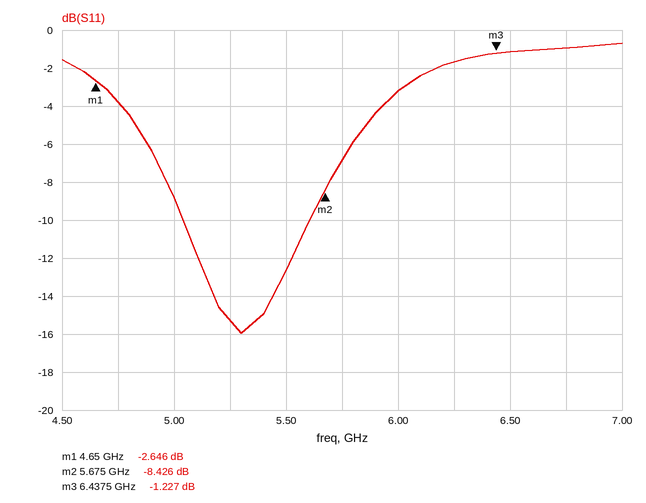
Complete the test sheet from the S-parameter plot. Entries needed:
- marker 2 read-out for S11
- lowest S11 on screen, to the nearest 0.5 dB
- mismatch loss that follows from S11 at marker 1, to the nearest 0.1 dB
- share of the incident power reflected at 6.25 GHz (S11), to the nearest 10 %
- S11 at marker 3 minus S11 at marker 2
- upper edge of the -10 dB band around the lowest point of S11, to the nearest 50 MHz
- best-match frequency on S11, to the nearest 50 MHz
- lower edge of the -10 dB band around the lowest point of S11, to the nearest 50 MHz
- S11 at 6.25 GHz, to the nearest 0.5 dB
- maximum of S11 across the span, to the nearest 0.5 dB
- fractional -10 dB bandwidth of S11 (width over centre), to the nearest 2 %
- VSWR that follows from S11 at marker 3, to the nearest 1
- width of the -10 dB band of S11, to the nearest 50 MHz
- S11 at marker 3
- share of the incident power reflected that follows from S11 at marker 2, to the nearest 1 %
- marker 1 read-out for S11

-8.426 dB
-16.0 dB
3.4 dB
70 %
7.199 dB
5.60 GHz
5.30 GHz
5.05 GHz
-1.5 dB
-0.5 dB
10 %
14
550 MHz
-1.227 dB
14 %
-2.646 dB
